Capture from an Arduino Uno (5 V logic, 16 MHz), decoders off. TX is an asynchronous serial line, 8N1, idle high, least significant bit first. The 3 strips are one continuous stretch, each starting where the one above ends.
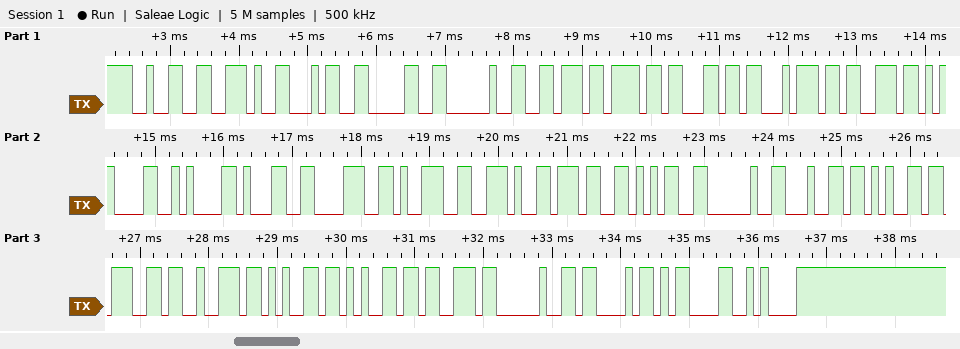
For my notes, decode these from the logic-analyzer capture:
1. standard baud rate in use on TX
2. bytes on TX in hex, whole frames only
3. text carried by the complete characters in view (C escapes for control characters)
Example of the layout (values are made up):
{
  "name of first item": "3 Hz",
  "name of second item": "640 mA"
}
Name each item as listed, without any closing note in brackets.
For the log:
{
  "standard baud rate in use on TX": "9600 baud",
  "bytes on TX in hex, whole frames only": "32 2E 34 30 20 76 6F 6C 74 73 0D 0A 31 38 39 2E 37 35 20 64 65 67 72 65 65 73 20 43 0D 0A",
  "text carried by the complete characters in view": "\"2.40 volts\\r\\n189.75 degrees C\\r\\n\""
}
